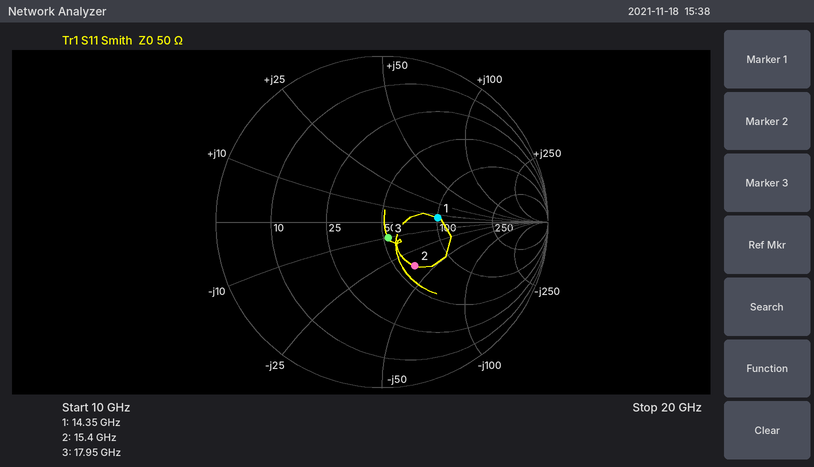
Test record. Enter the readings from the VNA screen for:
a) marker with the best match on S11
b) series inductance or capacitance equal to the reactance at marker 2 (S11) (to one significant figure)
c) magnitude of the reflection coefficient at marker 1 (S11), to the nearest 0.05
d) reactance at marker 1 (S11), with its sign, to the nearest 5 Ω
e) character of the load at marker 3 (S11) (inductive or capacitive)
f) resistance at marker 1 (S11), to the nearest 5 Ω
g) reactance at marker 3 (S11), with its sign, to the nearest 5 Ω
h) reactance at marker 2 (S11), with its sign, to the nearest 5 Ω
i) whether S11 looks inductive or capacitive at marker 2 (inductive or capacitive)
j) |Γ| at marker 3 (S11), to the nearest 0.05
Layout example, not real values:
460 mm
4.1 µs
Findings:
marker 3
300 fF
0.35
+5 Ω
capacitive
100 Ω
-10 Ω
-35 Ω
capacitive
0.10
